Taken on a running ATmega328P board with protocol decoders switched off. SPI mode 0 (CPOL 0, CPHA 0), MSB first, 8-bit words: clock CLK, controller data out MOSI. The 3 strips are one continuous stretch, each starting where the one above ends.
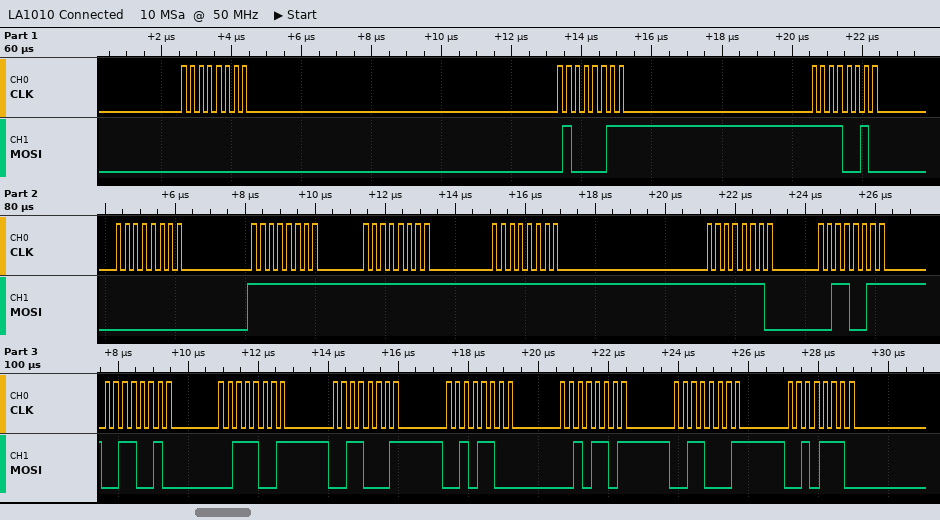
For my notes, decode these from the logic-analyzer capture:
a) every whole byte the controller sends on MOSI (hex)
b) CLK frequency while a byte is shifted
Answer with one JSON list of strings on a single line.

["00 43 F2 00 FF FF FF FE 33 32 39 31 2C 2D 31 2E", "4 MHz"]
